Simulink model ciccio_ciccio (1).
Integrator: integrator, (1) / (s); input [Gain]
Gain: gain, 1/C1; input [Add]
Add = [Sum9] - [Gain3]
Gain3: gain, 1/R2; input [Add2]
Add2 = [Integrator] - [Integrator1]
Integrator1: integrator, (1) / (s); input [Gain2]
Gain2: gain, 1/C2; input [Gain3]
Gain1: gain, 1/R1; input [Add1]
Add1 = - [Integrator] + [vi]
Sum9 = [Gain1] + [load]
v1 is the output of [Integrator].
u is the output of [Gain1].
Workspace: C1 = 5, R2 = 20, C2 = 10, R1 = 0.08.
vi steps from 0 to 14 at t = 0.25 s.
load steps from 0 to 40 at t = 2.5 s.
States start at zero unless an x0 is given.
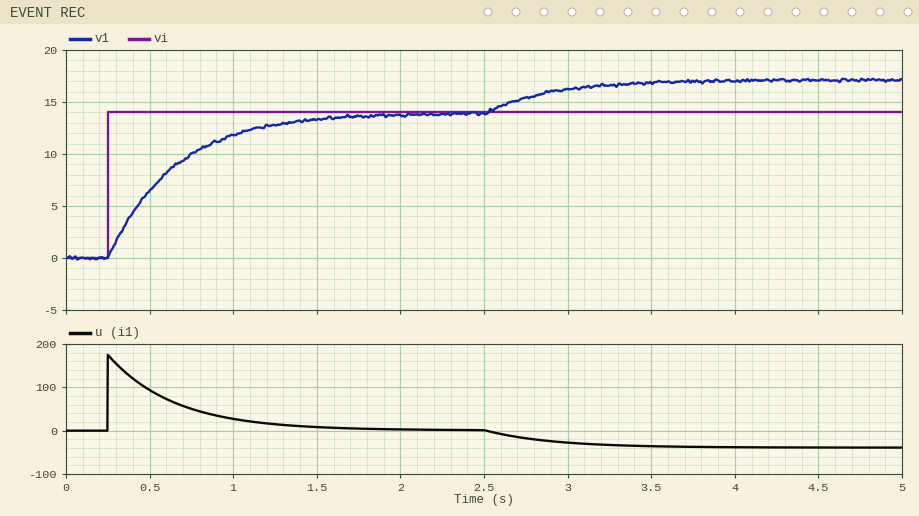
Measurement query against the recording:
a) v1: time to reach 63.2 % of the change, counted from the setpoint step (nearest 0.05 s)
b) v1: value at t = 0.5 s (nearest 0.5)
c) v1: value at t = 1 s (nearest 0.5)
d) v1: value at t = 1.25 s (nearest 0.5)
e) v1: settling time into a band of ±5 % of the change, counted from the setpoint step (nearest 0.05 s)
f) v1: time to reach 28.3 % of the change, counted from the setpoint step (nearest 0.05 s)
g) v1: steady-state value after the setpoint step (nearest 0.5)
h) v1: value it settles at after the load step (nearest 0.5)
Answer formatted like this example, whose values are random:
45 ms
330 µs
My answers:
0.40 s
6.5
12.0
13.0
1.20 s
0.15 s
14.0
17.0
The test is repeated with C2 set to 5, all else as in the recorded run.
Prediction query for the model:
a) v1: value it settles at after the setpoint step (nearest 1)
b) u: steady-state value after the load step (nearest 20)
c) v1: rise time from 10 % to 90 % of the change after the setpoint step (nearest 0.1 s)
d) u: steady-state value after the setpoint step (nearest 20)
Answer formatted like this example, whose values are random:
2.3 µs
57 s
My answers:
14
-40
0.9 s
0
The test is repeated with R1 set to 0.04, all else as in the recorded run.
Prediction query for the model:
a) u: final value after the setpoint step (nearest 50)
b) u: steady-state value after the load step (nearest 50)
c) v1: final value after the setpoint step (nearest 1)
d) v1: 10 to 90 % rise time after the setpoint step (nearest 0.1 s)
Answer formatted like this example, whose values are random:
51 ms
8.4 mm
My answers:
0
-50
14
0.4 s
